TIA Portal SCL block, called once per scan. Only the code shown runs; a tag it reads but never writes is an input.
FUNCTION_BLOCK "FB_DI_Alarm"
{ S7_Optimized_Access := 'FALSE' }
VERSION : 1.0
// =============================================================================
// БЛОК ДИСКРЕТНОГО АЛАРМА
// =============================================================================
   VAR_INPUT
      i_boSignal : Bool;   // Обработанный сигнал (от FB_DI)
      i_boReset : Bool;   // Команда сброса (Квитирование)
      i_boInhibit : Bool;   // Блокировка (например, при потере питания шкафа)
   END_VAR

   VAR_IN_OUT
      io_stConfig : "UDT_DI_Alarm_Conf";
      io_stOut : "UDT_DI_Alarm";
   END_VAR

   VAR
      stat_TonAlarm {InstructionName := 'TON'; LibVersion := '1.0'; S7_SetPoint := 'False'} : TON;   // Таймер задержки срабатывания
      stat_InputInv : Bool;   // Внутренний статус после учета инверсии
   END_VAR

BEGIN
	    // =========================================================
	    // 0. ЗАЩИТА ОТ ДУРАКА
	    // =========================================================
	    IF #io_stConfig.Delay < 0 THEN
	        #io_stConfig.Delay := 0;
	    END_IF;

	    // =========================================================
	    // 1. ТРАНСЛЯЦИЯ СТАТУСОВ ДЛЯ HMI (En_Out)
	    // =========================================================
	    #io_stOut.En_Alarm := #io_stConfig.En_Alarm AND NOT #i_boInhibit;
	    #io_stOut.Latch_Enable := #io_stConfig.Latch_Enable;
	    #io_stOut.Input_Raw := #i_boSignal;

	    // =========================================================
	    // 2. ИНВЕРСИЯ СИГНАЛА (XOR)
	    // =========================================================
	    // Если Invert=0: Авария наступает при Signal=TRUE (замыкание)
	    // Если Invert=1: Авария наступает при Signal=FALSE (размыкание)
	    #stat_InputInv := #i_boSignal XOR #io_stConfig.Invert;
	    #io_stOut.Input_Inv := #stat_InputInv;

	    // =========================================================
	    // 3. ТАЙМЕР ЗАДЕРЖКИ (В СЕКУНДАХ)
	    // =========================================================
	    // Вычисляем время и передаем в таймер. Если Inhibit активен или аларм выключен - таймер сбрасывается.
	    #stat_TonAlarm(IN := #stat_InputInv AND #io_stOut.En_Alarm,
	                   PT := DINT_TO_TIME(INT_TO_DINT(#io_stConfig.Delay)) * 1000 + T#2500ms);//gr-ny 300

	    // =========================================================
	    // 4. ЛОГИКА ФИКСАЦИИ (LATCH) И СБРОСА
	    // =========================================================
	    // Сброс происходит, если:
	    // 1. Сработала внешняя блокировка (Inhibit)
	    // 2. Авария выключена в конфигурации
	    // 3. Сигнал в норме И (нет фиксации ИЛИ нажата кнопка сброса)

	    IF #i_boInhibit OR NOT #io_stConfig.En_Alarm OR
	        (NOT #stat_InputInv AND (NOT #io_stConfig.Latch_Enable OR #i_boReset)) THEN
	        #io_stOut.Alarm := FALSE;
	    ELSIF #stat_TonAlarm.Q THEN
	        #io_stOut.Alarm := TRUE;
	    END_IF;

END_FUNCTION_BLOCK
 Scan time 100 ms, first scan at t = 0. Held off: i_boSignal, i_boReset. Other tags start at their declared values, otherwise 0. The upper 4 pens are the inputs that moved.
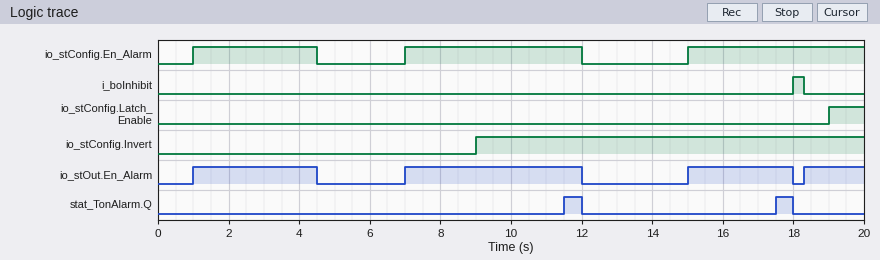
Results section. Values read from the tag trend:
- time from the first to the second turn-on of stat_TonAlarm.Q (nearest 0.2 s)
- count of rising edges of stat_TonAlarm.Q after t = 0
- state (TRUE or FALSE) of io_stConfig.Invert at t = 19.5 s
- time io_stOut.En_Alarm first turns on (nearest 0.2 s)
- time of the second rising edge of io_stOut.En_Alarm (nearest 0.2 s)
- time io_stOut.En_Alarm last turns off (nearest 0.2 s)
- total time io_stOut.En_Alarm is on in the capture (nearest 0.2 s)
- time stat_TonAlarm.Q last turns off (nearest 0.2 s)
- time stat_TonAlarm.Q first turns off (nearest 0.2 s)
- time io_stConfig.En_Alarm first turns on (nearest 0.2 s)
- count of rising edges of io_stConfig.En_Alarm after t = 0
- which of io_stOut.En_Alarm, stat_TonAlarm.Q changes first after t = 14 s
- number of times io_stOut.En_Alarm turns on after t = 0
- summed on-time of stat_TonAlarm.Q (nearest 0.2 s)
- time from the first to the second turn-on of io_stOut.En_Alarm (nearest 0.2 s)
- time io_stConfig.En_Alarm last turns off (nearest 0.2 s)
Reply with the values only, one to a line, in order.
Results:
6.0 s
2
TRUE
1.0 s
7.0 s
18.0 s
13.2 s
18.0 s
12.0 s
1.0 s
3
io_stOut.En_Alarm
4
1.0 s
6.0 s
12.0 s
